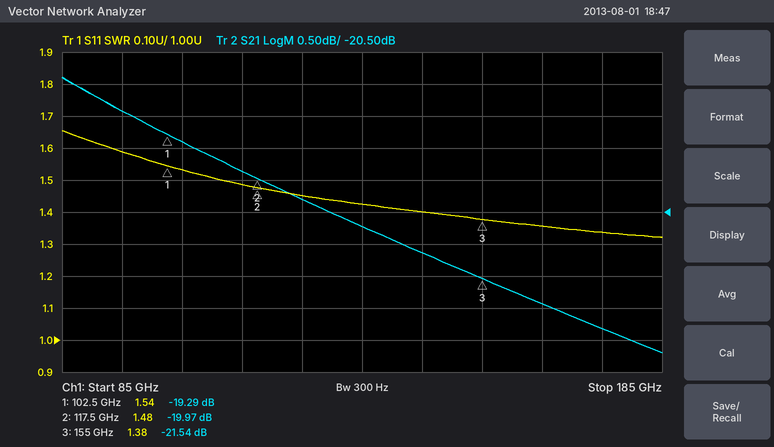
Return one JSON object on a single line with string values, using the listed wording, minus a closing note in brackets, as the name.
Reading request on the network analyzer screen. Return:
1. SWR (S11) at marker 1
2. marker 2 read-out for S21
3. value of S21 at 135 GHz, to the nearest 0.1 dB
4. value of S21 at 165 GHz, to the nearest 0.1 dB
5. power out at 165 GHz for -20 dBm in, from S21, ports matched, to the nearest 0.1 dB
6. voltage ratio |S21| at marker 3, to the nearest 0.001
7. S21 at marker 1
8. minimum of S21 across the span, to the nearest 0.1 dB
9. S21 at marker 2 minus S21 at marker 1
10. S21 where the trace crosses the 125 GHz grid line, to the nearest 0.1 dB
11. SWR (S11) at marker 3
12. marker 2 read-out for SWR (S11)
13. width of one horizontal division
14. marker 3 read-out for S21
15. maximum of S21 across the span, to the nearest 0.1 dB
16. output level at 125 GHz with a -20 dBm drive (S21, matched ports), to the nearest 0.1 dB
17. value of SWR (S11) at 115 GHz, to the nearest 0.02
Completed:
{"SWR (S11) at marker 1": "1.54", "marker 2 read-out for S21": "-19.97 dB", "value of S21 at 135 GHz, to the nearest 0.1 dB": "-20.7 dB", "value of S21 at 165 GHz, to the nearest 0.1 dB": "-21.9 dB", "power out at 165 GHz for -20 dBm in, from S21, ports matched, to the nearest 0.1 dB": "-41.9 dBm", "voltage ratio |S21| at marker 3, to the nearest 0.001": "0.084", "S21 at marker 1": "-19.29 dB", "minimum of S21 across the span, to the nearest 0.1 dB": "-22.7 dB", "S21 at marker 2 minus S21 at marker 1": "-0.68 dB", "S21 where the trace crosses the 125 GHz grid line, to the nearest 0.1 dB": "-20.3 dB", "SWR (S11) at marker 3": "1.38", "marker 2 read-out for SWR": "1.48", "width of one horizontal division": "10 GHz", "marker 3 read-out for S21": "-21.54 dB", "maximum of S21 across the span, to the nearest 0.1 dB": "-18.4 dB", "output level at 125 GHz with a -20 dBm drive (S21, matched ports), to the nearest 0.1 dB": "-40.3 dBm", "value of SWR (S11) at 115 GHz, to the nearest 0.02": "1.48"}
